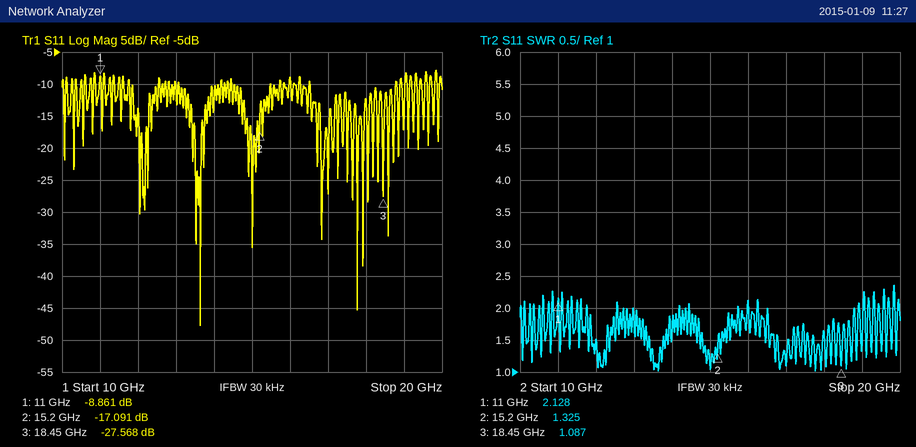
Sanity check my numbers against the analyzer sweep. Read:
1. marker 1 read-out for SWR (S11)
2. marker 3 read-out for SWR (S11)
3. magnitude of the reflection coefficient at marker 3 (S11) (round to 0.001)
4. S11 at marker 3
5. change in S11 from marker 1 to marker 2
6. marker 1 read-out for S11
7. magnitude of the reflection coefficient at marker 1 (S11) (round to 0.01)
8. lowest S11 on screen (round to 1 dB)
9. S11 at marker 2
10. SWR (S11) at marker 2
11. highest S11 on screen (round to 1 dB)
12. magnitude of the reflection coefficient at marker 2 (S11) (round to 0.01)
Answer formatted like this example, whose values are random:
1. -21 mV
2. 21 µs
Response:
1. 2.128
2. 1.087
3. 0.042
4. -27.568 dB
5. -8.230 dB
6. -8.861 dB
7. 0.36
8. -48 dB
9. -17.091 dB
10. 1.325
11. -8 dB
12. 0.14
